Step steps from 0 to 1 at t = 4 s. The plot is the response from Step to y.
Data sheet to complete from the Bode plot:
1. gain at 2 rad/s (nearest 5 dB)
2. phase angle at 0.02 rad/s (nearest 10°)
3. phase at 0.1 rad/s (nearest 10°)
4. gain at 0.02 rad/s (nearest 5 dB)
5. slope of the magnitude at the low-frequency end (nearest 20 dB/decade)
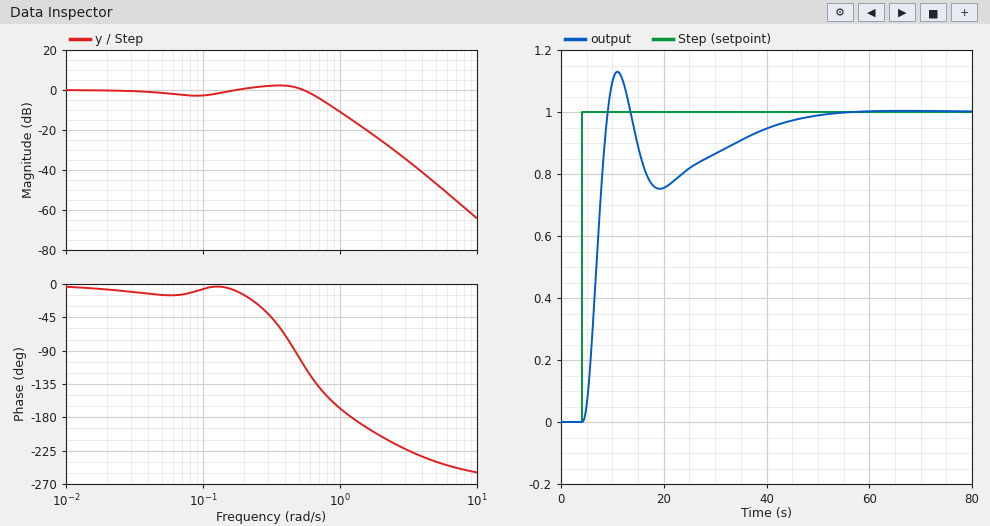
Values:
-25 dB
-10°
-10°
0 dB
0 dB/decade
